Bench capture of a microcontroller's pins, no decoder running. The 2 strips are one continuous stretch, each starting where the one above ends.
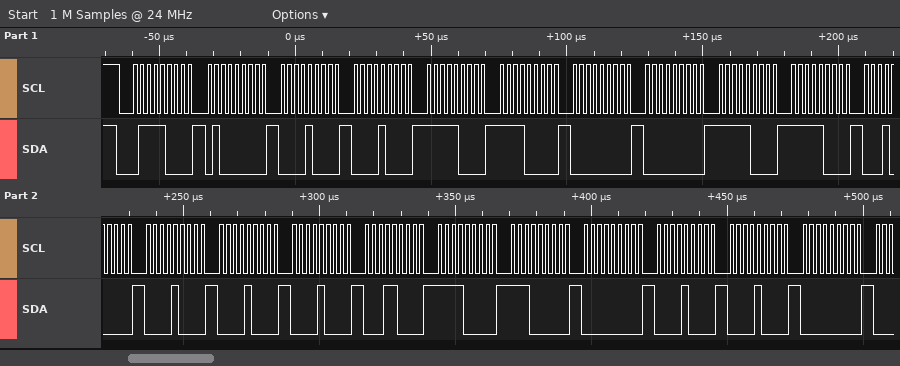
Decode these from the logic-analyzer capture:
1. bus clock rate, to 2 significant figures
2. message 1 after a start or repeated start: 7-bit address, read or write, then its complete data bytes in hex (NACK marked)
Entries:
400 kHz
0x3C write: 40 08 08 F8 F0 00 00 F8 F8 10 08 08 08 18 F0 E0 00 08 08 00
